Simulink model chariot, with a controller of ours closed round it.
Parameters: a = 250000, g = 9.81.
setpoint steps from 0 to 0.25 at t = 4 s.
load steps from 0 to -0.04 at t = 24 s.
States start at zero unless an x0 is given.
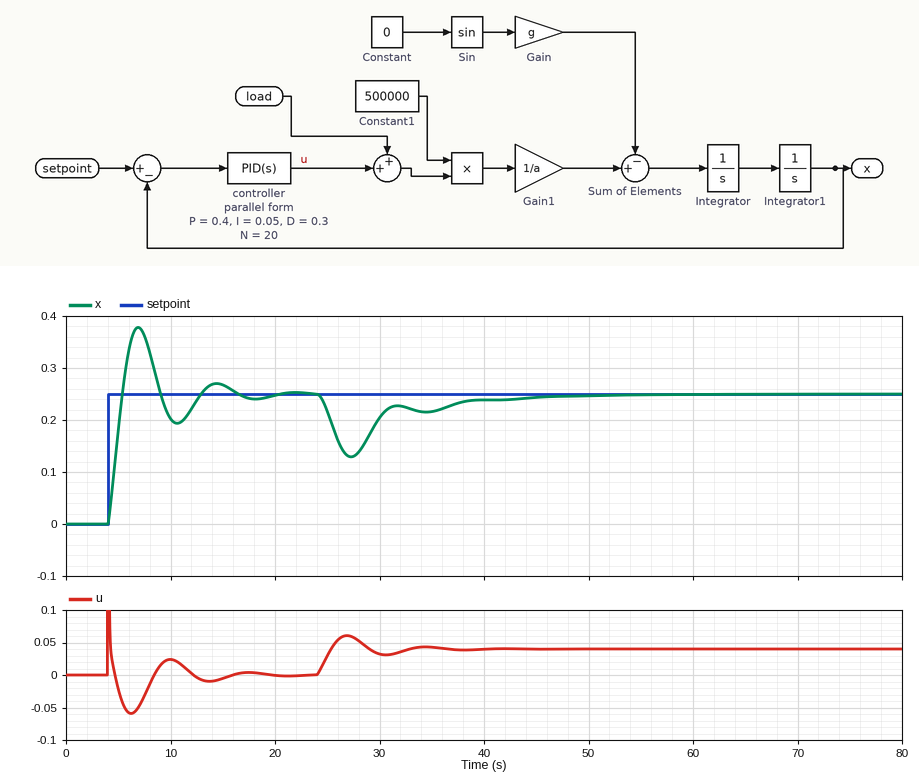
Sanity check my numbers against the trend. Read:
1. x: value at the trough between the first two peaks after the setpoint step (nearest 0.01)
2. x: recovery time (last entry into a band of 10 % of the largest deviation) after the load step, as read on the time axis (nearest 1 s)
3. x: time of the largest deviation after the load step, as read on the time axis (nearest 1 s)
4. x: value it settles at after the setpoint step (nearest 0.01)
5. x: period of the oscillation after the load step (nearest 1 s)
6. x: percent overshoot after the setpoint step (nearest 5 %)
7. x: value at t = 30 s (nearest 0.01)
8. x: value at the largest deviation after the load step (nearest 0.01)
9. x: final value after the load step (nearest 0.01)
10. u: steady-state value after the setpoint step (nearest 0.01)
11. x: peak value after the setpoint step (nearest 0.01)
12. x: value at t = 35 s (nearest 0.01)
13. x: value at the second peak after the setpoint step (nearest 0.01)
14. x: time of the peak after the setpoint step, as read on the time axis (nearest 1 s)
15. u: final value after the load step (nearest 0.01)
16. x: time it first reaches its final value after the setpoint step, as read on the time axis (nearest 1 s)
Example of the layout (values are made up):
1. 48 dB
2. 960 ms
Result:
1. 0.19
2. 39 s
3. 27 s
4. 0.25
5. 7 s
6. 50 %
7. 0.20
8. 0.13
9. 0.25
10. 0.00
11. 0.38
12. 0.22
13. 0.27
14. 7 s
15. 0.04
16. 5 s
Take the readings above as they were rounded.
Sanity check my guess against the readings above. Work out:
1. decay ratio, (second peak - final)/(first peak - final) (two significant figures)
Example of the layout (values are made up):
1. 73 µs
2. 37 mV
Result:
1. 0.15
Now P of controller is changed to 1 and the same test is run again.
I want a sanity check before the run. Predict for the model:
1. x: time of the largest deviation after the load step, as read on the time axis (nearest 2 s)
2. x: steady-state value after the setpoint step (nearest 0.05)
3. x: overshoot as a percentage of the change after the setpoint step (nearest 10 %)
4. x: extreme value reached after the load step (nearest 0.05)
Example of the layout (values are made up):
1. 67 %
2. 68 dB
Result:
1. 26 s
2. 0.25
3. 60 %
4. 0.20
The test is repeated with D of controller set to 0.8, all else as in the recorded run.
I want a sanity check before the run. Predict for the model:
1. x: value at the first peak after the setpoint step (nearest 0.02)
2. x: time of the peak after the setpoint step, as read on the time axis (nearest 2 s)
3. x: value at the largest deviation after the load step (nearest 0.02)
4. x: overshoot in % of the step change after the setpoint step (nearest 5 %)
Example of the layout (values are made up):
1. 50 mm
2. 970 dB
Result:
1. 0.30
2. 6 s
3. 0.16
4. 20 %
